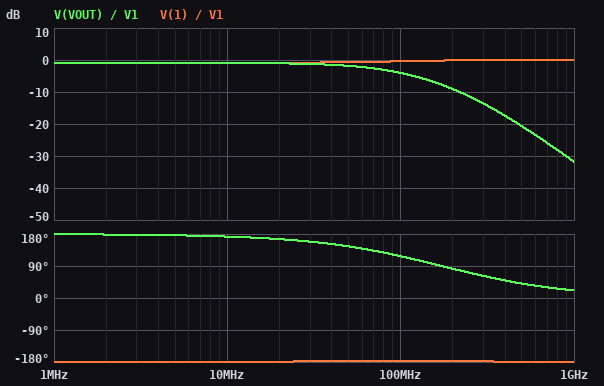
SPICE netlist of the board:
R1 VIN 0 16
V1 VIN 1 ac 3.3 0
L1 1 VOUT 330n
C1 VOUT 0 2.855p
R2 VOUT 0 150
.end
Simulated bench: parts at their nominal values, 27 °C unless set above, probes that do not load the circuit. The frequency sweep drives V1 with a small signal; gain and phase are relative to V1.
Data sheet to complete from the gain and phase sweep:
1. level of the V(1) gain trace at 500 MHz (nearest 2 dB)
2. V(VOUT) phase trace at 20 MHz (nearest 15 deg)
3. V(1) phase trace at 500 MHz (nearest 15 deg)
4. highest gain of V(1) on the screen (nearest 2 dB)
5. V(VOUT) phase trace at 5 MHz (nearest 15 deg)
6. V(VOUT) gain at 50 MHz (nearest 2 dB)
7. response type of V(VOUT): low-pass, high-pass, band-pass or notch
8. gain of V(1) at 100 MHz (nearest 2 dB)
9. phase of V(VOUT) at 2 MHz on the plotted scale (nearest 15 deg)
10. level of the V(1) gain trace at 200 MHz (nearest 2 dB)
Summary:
0 dB
165 deg
-180 deg
0 dB
180 deg
-2 dB
low-pass
0 dB
180 deg
0 dB
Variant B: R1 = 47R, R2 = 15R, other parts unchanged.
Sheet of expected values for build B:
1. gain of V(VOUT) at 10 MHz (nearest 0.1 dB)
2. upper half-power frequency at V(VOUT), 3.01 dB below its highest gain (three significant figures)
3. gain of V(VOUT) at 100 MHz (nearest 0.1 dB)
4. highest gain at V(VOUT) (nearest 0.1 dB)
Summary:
-12.8 dB
30.0 MHz
-23.2 dB
-12.3 dB
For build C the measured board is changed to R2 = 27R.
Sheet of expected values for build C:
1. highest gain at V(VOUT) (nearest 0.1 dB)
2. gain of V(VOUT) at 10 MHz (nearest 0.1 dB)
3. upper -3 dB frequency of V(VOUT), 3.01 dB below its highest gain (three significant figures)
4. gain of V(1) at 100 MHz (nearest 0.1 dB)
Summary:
-4.0 dB
-4.9 dB
20.9 MHz
-0.1 dB
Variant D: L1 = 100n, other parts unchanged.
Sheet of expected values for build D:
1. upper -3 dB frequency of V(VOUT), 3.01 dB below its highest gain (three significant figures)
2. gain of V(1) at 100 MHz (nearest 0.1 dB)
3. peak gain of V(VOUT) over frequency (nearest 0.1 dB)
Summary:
340 MHz
-0.9 dB
-0.7 dB
